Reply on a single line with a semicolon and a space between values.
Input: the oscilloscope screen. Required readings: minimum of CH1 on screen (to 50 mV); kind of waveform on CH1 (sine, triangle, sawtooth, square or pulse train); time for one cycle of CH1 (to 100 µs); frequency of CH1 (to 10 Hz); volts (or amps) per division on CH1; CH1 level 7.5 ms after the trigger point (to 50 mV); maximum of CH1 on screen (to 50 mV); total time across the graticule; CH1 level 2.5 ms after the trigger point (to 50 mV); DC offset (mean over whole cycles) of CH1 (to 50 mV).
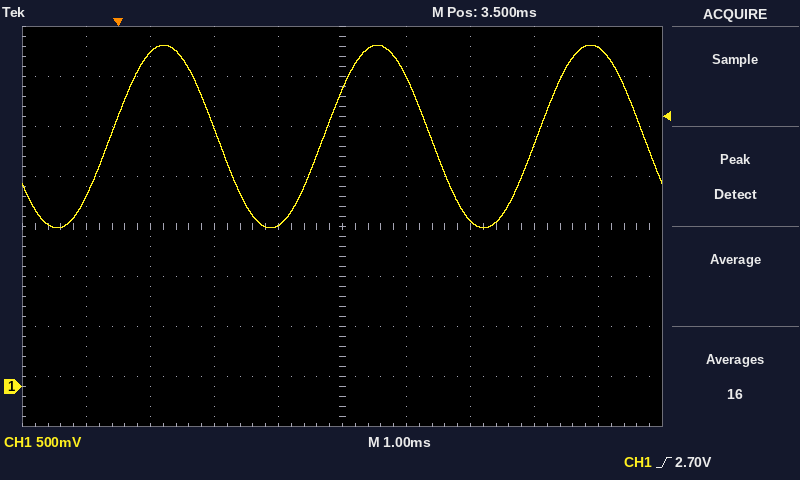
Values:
1.60 V; sine; 3.3 ms; 300 Hz; 500 mV; 3.40 V; 3.40 V; 10 ms; 1.60 V; 2.50 V
